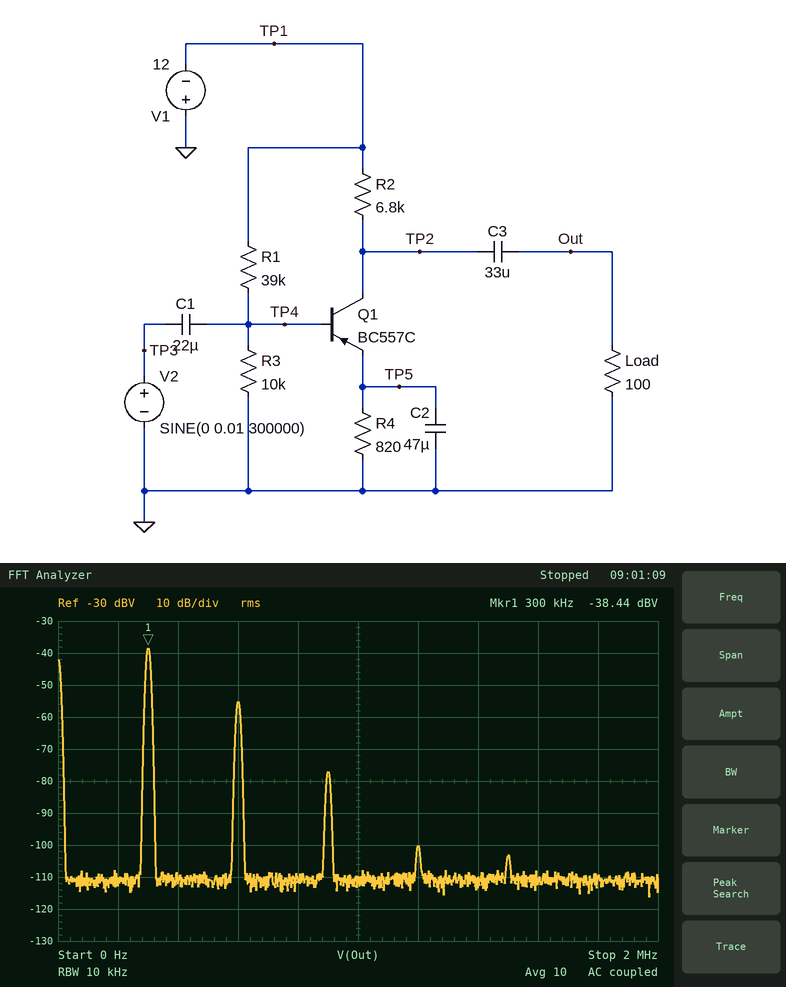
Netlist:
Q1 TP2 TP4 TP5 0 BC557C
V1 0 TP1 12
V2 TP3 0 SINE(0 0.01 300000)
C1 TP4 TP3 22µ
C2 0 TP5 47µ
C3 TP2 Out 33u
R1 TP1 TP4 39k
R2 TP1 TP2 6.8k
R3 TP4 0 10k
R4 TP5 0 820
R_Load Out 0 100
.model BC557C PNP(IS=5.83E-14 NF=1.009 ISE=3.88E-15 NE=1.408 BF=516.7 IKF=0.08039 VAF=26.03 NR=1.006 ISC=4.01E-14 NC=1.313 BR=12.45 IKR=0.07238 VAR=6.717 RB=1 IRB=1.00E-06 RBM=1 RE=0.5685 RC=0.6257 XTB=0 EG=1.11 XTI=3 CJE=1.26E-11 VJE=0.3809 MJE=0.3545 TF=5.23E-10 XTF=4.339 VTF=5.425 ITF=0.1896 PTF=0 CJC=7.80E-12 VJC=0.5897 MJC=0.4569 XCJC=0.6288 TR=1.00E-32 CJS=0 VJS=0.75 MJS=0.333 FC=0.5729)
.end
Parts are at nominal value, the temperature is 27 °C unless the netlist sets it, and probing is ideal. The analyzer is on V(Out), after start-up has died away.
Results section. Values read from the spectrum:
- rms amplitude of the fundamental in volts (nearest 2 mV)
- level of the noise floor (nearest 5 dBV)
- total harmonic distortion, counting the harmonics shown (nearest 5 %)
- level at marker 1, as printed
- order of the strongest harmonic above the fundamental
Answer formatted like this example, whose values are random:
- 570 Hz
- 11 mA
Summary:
- 12 mV
- -110 dBV
- 15 %
- -38.44 dBV
- 2
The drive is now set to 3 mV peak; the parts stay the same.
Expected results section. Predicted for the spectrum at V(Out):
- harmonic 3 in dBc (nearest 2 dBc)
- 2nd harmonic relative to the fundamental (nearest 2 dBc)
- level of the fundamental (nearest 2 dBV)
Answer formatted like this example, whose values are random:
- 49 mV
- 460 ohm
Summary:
- -58 dBc
- -26 dBc
- -50 dBV
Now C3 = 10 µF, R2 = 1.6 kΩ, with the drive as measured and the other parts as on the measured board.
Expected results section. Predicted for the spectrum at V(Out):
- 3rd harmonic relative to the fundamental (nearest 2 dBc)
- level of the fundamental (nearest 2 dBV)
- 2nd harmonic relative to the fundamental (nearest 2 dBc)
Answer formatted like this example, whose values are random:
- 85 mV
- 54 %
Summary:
- -48 dBc
- -26 dBV
- -22 dBc
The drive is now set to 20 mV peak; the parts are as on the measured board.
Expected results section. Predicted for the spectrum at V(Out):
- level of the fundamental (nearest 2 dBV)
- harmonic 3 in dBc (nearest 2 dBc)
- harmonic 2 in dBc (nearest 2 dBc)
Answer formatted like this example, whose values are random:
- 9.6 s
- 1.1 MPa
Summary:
- -32 dBV
- -34 dBc
- -12 dBc
